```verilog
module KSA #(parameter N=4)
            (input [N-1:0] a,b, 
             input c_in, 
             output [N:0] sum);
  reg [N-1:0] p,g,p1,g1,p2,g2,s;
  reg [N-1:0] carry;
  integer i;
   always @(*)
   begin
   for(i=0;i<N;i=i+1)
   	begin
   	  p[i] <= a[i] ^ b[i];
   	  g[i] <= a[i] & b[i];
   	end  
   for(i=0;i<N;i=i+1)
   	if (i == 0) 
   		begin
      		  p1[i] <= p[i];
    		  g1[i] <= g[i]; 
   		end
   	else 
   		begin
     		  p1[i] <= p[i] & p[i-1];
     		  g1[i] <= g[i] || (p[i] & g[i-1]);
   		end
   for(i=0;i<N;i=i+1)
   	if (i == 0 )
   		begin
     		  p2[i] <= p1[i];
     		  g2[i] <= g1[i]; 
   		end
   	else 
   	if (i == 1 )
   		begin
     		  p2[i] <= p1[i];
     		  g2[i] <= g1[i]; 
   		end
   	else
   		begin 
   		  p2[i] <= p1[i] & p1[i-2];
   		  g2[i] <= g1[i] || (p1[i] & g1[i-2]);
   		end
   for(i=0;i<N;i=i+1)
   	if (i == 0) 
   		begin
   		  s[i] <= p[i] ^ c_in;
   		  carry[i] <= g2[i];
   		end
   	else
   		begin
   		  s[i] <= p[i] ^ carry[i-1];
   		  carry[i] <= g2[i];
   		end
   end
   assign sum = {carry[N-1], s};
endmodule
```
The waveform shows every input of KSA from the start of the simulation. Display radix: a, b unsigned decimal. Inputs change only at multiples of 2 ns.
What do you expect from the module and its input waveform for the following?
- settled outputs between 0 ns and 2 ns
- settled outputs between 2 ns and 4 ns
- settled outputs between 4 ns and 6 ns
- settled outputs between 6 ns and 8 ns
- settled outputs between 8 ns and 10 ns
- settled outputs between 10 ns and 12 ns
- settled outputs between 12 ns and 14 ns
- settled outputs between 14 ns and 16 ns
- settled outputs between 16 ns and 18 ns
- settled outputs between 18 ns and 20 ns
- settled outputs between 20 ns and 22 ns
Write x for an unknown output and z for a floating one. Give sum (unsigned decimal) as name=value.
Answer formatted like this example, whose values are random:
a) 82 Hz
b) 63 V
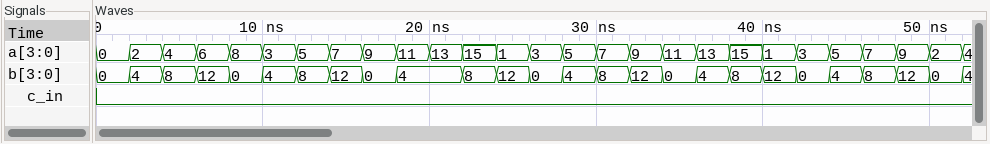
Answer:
a) sum=0
b) sum=6
c) sum=12
d) sum=18
e) sum=8
f) sum=7
g) sum=13
h) sum=19
i) sum=9
j) sum=15
k) sum=17
